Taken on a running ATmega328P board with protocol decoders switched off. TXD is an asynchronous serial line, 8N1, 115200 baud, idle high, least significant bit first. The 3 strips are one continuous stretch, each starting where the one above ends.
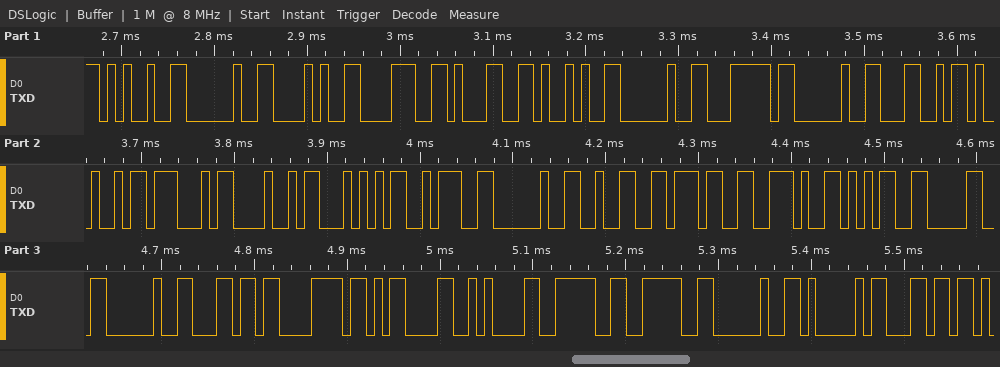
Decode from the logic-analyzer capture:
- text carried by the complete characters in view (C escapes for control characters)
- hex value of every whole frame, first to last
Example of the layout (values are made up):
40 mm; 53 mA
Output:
"% (81) | LIGHT: 27.50 lx\r\n>> Al"; 0x25 0x20 0x28 0x38 0x31 0x29 0x20 0x7C 0x20 0x4C 0x49 0x47 0x48 0x54 0x3A 0x20 0x32 0x37 0x2E 0x35 0x30 0x20 0x6C 0x78 0x0D 0x0A 0x3E 0x3E 0x20 0x41 0x6C
